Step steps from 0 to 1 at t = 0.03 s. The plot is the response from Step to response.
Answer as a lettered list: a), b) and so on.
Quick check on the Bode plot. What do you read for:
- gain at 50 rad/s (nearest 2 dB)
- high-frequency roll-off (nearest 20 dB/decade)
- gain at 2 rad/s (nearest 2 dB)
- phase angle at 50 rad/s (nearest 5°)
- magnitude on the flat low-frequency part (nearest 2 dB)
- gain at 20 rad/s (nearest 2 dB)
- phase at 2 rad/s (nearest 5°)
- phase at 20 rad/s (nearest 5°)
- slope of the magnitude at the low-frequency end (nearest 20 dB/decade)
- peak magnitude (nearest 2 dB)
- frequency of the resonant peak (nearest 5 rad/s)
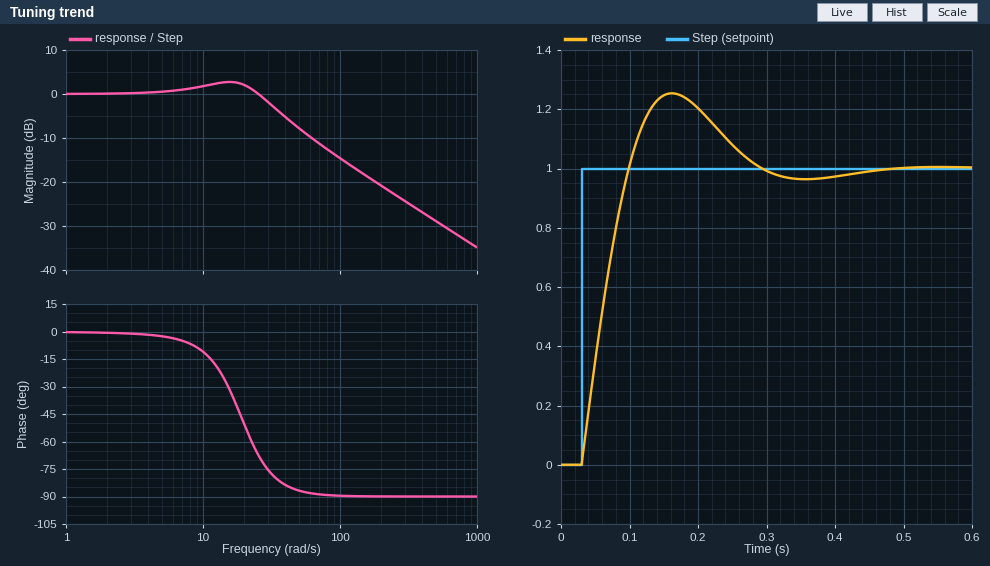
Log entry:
a) -8 dB
b) -20 dB/decade
c) 0 dB
d) -85°
e) 0 dB
f) 2 dB
g) 0°
h) -50°
i) 0 dB/decade
j) 2 dB
k) 15 rad/s
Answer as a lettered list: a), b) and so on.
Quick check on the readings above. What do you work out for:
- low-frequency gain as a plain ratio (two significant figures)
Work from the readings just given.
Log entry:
a) 1.0
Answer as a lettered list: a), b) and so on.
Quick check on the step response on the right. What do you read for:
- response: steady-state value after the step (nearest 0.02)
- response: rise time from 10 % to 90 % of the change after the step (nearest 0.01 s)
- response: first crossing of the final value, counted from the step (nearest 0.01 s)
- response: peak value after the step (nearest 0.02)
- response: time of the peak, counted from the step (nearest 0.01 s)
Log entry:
a) 1.00
b) 0.05 s
c) 0.07 s
d) 1.26
e) 0.13 s
